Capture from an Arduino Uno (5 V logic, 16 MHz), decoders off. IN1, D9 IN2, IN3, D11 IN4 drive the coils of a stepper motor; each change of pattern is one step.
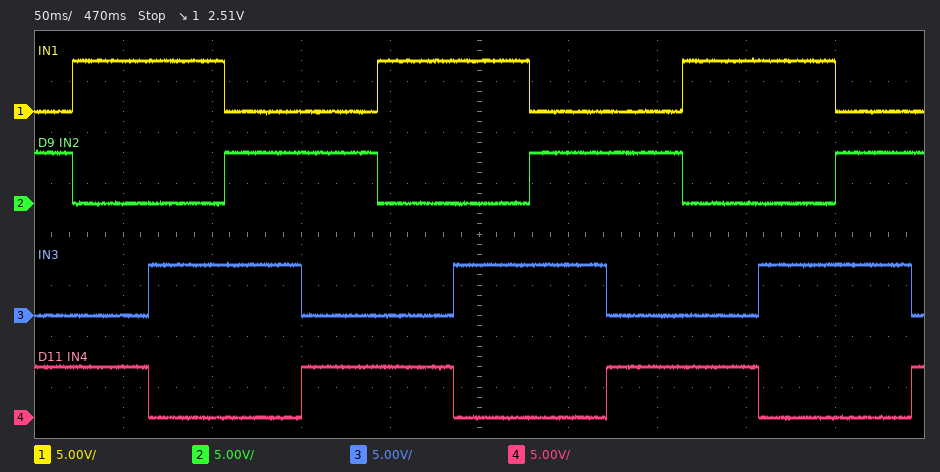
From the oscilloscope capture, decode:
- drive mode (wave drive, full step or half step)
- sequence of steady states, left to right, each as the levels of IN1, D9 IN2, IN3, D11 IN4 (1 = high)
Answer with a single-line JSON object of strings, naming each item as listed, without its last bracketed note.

{"drive mode": "full step", "sequence of steady states, left to right, each as the levels of IN1, D9 IN2, IN3, D11 IN4": "0101 1001 1010 0110 0101 1001 1010 0110 0101 1001 1010 0110 0101"}
